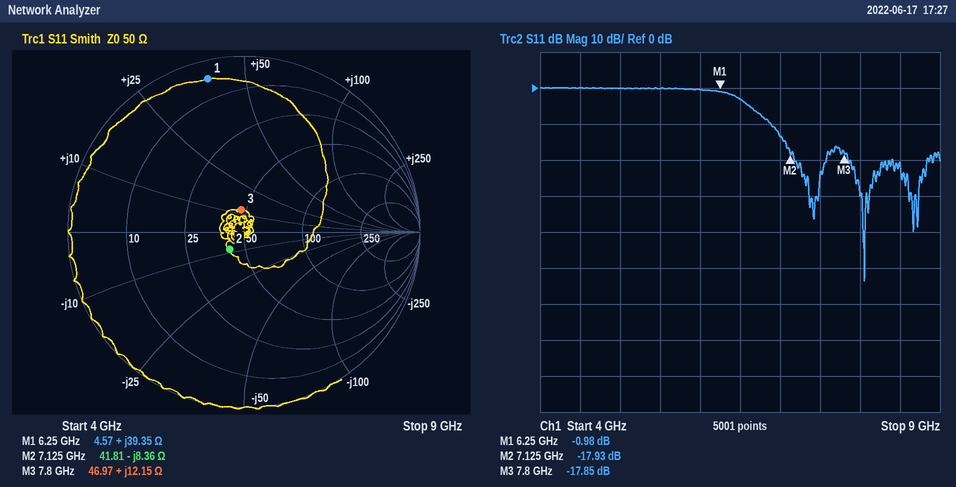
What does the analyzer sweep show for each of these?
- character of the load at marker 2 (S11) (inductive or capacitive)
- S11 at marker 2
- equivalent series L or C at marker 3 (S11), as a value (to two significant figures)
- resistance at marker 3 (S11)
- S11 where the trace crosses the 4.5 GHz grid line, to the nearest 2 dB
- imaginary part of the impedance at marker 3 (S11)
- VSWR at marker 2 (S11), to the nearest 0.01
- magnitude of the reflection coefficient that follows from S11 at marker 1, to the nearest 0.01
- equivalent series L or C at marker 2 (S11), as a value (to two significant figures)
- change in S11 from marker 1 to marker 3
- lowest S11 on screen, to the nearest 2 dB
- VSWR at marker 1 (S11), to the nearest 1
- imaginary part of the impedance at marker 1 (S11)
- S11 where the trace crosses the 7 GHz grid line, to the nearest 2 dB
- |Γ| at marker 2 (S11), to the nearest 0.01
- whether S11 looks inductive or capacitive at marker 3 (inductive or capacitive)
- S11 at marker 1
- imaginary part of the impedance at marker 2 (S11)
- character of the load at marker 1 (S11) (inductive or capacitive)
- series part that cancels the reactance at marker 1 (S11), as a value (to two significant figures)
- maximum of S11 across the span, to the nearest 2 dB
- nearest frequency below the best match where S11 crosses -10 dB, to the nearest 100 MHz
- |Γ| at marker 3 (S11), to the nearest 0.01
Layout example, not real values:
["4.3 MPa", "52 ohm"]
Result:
["capacitive", "-17.93 dB", "250 pH", "46.97 Ω", "0 dB", "+12.15 Ω", "1.29", "0.89", "2.7 pF", "-16.87 dB", "-54 dB", "18", "+39.35 Ω", "-14 dB", "0.13", "inductive", "-0.98 dB", "-8.36 Ω", "inductive", "650 fF", "0 dB", "6.9 GHz", "0.13"]
